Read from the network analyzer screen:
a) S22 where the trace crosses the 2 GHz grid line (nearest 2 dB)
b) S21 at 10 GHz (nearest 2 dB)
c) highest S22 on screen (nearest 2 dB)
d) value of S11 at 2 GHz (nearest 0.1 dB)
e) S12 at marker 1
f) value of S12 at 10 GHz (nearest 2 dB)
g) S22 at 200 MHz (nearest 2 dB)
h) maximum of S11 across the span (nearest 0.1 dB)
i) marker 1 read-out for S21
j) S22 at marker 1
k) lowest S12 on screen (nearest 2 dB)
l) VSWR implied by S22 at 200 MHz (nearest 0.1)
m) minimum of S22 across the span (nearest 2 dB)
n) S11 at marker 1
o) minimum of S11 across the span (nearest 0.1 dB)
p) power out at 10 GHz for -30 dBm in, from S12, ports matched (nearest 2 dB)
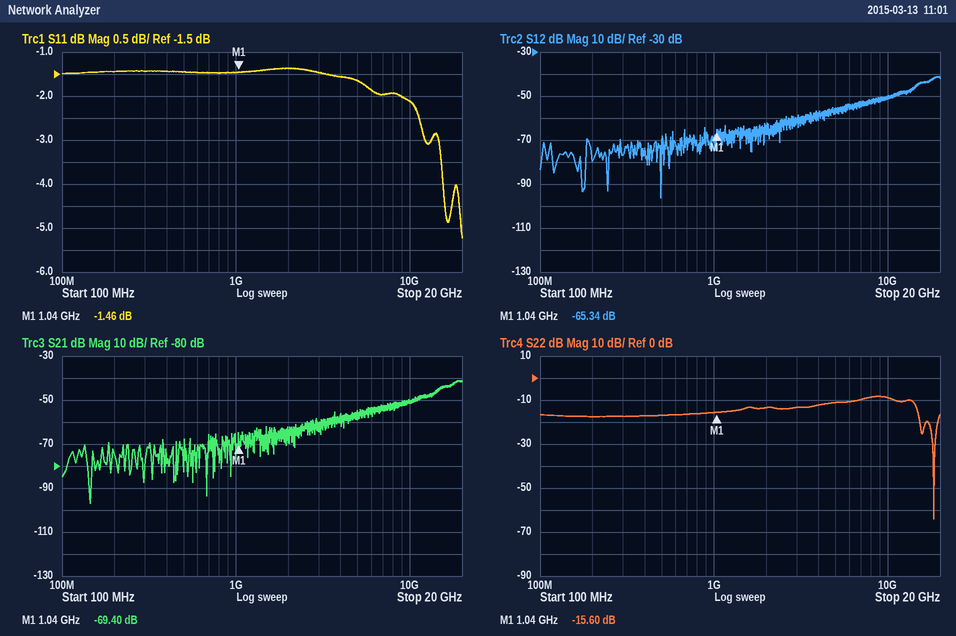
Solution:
-14 dB
-50 dB
-8 dB
-1.4 dB
-65.34 dB
-50 dB
-18 dB
-1.4 dB
-69.40 dB
-15.60 dB
-96 dB
1.3
-64 dB
-1.46 dB
-5.2 dB
-80 dBm
